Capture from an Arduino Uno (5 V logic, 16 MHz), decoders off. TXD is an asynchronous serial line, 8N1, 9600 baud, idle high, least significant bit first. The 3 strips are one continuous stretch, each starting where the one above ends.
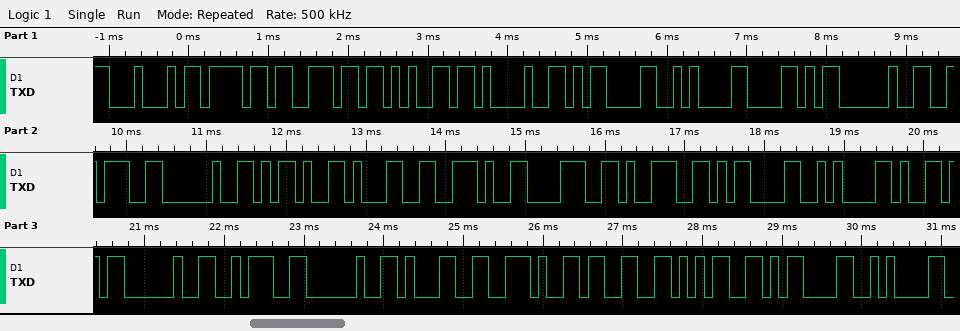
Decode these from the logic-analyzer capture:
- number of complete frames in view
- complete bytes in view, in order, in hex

28
0x44 0x6F 0x6E 0x65 0x21 0x0D 0x0A 0x58 0x20 0x3A 0x20 0x2D 0x31 0x2E 0x38 0x39 0x0D 0x0A 0x59 0x20 0x3A 0x20 0x31 0x2E 0x33 0x35 0x0D 0x0A
